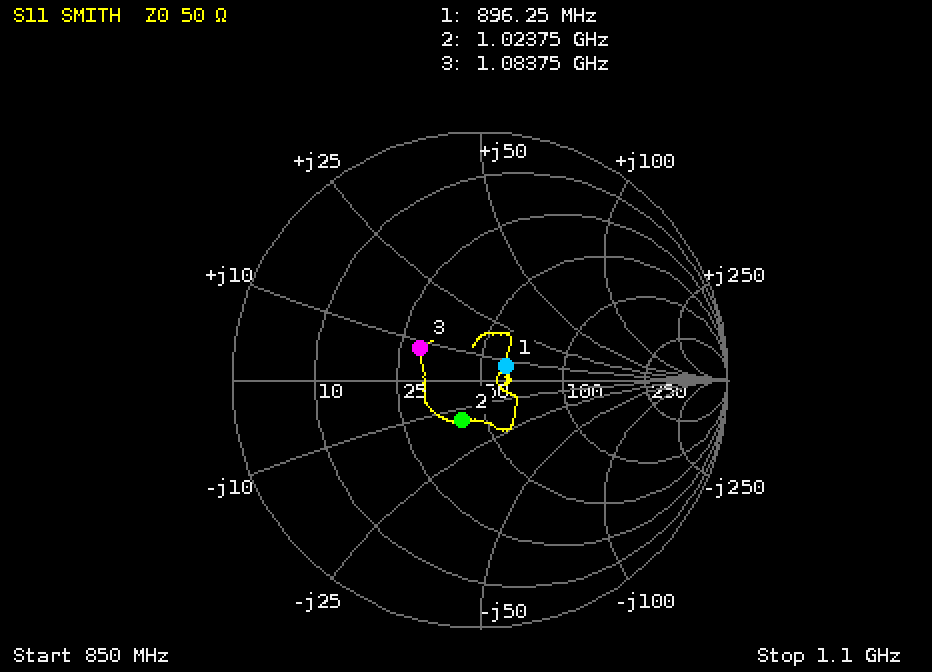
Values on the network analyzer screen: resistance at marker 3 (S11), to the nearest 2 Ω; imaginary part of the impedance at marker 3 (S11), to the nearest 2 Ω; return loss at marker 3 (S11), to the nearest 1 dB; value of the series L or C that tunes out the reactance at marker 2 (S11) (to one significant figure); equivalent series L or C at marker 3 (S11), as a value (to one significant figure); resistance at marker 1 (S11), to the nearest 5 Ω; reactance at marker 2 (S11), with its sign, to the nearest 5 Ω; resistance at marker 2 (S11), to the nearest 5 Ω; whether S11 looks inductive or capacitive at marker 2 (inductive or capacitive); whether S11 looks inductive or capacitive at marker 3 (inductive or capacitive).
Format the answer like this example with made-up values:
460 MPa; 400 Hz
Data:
30 Ω; +8 Ω; 11 dB; 2 nH; 1 nH; 60 Ω; -15 Ω; 40 Ω; capacitive; inductive
